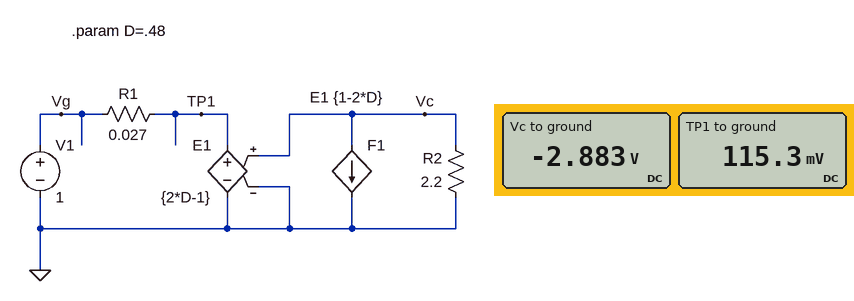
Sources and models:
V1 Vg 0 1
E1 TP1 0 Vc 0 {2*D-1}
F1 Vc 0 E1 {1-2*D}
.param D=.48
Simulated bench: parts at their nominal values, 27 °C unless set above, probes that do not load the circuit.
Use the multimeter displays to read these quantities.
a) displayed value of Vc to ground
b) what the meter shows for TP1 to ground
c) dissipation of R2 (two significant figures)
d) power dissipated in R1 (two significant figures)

-2.883 V
115.3 mV
3.8 W
29 W
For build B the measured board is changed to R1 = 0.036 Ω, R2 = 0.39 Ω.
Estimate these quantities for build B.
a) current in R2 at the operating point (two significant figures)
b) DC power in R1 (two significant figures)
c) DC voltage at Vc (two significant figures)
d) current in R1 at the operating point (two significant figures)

1.1 A
27 W
-430 mV
27 A
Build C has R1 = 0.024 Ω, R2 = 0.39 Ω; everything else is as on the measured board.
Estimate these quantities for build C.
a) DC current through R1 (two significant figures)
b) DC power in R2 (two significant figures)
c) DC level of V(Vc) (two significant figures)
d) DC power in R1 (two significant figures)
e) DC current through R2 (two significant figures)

41 A
1.0 W
-630 mV
40 W
1.6 A
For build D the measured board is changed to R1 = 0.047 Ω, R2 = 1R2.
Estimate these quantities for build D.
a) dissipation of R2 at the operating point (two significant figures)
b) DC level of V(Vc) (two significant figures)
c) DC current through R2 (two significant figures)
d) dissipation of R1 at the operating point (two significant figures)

800 mW
-980 mV
820 mA
20 W
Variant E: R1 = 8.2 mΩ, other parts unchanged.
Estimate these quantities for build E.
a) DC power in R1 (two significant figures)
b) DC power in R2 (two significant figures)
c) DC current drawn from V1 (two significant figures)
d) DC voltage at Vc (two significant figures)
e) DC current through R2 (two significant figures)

60 W
26 W
85 A
-7.5 V
3.4 A
